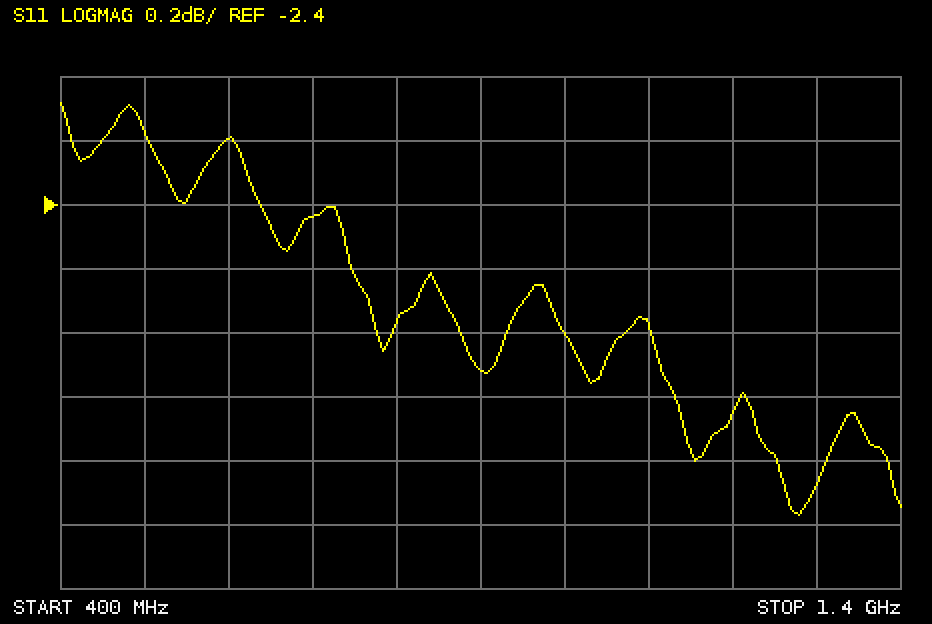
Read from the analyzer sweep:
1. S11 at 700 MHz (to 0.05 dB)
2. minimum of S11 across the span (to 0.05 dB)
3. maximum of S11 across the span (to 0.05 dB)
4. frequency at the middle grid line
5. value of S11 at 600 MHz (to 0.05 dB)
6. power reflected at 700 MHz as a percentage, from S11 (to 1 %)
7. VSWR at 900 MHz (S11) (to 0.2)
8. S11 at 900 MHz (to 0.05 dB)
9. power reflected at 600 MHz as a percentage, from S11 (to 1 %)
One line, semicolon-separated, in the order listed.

-2.45 dB; -3.35 dB; -2.10 dB; 900 MHz; -2.20 dB; 57 %; 6.0; -2.90 dB; 60 %
